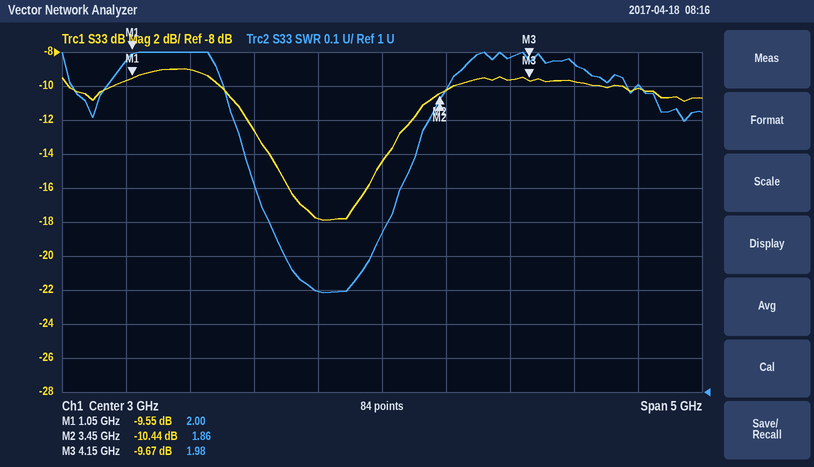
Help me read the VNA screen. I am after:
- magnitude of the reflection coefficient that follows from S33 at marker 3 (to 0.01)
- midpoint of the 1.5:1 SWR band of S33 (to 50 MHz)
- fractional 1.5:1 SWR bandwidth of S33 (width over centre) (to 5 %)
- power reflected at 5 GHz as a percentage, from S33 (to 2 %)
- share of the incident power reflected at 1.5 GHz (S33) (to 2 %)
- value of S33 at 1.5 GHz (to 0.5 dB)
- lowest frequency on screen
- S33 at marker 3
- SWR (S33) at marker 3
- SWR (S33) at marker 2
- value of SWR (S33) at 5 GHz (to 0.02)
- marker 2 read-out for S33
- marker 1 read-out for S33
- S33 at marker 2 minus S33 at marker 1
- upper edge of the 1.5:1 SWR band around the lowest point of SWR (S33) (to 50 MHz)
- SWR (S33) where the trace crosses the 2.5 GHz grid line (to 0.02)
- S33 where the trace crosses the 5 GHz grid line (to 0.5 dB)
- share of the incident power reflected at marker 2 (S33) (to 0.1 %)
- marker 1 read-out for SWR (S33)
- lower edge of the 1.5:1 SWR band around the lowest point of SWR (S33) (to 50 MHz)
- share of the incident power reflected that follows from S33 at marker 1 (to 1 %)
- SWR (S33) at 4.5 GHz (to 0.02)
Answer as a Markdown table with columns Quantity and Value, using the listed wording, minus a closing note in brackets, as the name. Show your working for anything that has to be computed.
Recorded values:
| Quantity | Value |
|---|---|
| magnitude of the reflection coefficient that follows from S33 at marker 3 | 10^(-9.67/20) ≈ 0.33 |
| midpoint of the 1.5:1 SWR band of S33 | 2.60 GHz |
| fractional 1.5:1 SWR bandwidth of S33 (width over centre) | 950 MHz / 2.575 GHz ≈ 36.9 %, so 35 % to the nearest 5 % |
| power reflected at 5 GHz as a percentage, from S33 | 10^(-10/10) ≈ 10 % |
| share of the incident power reflected at 1.5 GHz (S33) | 10^(-9/10) ≈ 12.6 %, so 12 % to the nearest 2 % |
| value of S33 at 1.5 GHz | -9.0 dB |
| lowest frequency on screen | 500 MHz |
| S33 at marker 3 | -9.67 dB |
| SWR (S33) at marker 3 | 1.98 |
| SWR (S33) at marker 2 | 1.86 |
| value of SWR (S33) at 5 GHz | 1.90 |
| marker 2 read-out for S33 | -10.44 dB |
| marker 1 read-out for S33 | -9.55 dB |
| S33 at marker 2 minus S33 at marker 1 | -10.44 − (-9.55) = -0.89 dB |
| upper edge of the 1.5:1 SWR band around the lowest point of SWR (S33) | 3.05 GHz |
| SWR (S33) where the trace crosses the 2.5 GHz grid line | 1.30 |
| S33 where the trace crosses the 5 GHz grid line | -10.0 dB |
| share of the incident power reflected at marker 2 (S33) | 10^(-10.44/10) ≈ 9.0 % |
| marker 1 read-out for SWR | 2.00 |
| lower edge of the 1.5:1 SWR band around the lowest point of SWR (S33) | 2.10 GHz |
| share of the incident power reflected that follows from S33 at marker 1 | 10^(-9.55/10) ≈ 11 % |
| SWR (S33) at 4.5 GHz | 1.96 |
